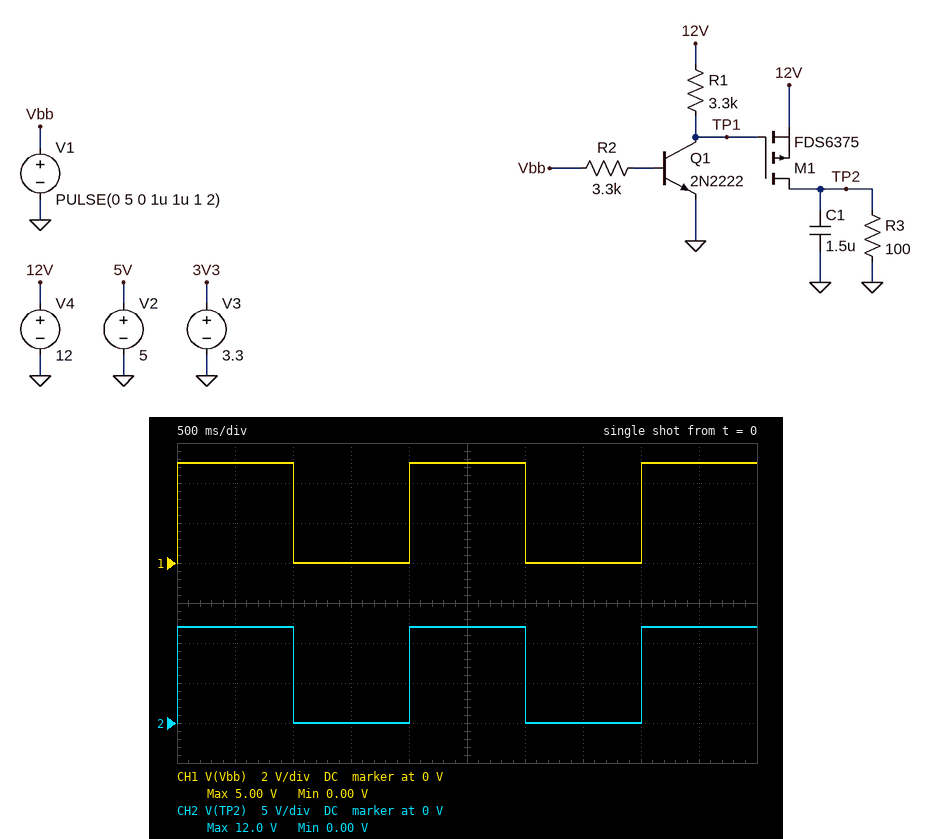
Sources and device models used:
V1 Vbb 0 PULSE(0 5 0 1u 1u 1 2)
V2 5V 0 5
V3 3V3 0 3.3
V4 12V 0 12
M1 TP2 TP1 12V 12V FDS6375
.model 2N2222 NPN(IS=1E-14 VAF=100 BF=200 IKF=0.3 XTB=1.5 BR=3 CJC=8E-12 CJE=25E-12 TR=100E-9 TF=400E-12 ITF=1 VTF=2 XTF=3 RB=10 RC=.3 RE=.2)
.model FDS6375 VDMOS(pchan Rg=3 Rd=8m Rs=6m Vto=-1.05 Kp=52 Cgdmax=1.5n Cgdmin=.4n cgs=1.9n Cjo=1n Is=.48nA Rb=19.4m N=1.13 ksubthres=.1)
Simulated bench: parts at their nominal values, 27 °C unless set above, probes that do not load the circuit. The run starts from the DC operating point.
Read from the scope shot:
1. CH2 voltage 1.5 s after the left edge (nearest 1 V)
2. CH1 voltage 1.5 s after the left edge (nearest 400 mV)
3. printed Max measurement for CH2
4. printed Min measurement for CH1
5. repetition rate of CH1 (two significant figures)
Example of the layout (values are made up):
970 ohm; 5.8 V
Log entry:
0 V; 0 V; 12.0 V; 0.00 V; 500 mHz
